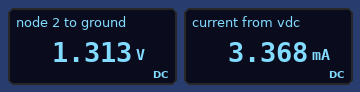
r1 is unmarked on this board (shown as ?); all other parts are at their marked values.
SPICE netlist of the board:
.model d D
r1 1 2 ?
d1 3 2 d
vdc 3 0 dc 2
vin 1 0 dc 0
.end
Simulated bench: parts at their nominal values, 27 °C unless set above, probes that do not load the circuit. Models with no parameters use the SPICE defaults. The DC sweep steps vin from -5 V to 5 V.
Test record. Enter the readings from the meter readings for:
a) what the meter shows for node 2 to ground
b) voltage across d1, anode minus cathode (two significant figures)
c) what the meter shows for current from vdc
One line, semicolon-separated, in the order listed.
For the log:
1.313 V; 690 mV; 3.368 mA
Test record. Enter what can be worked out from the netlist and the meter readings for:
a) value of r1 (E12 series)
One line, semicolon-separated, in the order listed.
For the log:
390 Ω
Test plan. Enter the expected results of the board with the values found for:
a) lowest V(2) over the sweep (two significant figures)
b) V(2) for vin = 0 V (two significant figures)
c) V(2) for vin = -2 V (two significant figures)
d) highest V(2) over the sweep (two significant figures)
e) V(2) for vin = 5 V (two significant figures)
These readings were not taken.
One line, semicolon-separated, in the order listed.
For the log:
1.3 V; 1.3 V; 1.3 V; 5.0 V; 5.0 V
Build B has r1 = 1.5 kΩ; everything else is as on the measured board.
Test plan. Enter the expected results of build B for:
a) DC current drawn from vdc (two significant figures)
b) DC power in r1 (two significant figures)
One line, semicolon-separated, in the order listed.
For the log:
900 µA; 1.2 mW
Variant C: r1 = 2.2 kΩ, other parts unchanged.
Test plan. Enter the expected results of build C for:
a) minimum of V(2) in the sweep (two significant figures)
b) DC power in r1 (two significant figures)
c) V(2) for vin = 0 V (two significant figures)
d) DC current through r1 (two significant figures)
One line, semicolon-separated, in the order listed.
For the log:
1.3 V; 840 µW; 1.4 V; 620 µA
